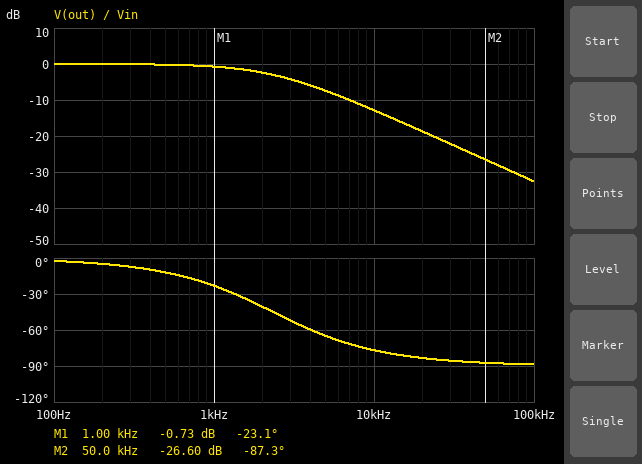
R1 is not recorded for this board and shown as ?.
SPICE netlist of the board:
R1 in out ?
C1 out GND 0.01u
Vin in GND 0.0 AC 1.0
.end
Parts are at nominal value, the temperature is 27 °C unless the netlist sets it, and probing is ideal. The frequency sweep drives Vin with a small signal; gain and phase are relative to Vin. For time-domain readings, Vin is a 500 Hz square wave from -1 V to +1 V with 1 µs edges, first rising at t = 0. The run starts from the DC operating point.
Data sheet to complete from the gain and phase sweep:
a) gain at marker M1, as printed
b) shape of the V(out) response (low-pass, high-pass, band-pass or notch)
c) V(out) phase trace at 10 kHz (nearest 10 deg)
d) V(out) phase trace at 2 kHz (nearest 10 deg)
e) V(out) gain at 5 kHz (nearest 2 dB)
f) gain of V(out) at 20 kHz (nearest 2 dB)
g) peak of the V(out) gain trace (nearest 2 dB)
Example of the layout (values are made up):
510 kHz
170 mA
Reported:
-0.73 dB
low-pass
-80 deg
-40 deg
-8 dB
-18 dB
0 dB
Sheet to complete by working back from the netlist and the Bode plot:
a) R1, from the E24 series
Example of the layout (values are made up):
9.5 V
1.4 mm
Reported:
6.8 kΩ
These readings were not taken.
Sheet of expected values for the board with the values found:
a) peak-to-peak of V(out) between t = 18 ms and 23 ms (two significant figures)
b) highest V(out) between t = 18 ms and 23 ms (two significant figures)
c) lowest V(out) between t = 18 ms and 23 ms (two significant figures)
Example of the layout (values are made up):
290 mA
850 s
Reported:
2.0 V
1.0 V
-1.0 V
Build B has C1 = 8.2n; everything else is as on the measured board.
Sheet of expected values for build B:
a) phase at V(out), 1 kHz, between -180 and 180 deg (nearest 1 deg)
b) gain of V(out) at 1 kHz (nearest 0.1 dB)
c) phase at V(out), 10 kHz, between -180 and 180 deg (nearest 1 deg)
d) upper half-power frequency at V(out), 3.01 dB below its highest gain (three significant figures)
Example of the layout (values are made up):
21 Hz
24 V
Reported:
-19 deg
-0.5 dB
-74 deg
2.85 kHz
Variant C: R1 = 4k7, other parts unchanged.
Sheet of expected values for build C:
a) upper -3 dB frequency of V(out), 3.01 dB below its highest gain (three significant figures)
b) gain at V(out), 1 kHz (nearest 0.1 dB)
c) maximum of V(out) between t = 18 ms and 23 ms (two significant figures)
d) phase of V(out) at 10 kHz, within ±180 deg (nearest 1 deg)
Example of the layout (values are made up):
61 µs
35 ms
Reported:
3.39 kHz
-0.4 dB
1.0 V
-71 deg
